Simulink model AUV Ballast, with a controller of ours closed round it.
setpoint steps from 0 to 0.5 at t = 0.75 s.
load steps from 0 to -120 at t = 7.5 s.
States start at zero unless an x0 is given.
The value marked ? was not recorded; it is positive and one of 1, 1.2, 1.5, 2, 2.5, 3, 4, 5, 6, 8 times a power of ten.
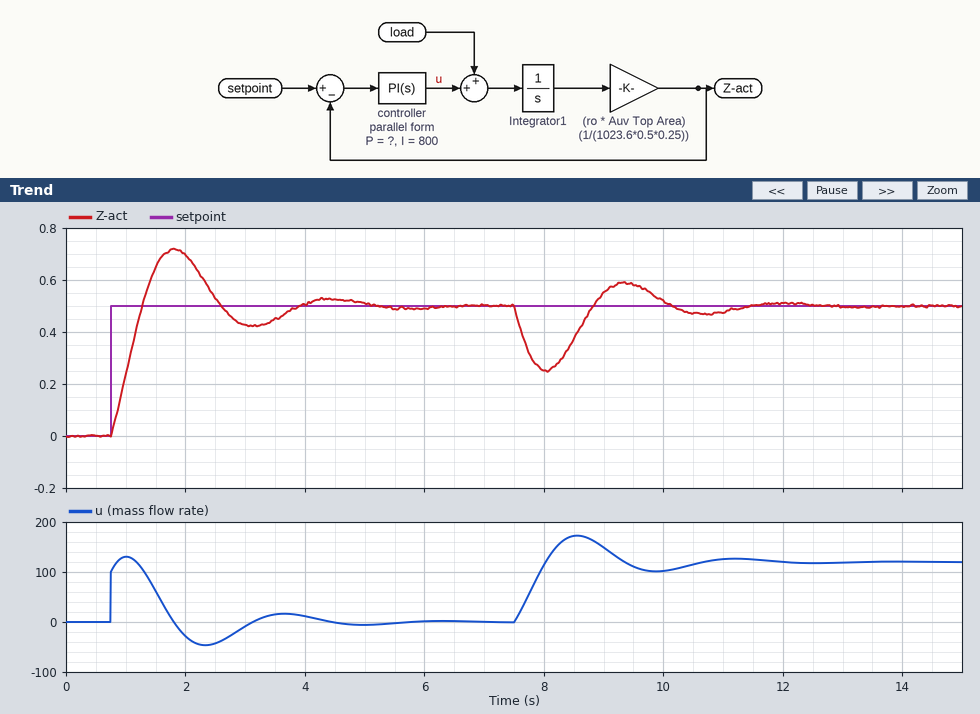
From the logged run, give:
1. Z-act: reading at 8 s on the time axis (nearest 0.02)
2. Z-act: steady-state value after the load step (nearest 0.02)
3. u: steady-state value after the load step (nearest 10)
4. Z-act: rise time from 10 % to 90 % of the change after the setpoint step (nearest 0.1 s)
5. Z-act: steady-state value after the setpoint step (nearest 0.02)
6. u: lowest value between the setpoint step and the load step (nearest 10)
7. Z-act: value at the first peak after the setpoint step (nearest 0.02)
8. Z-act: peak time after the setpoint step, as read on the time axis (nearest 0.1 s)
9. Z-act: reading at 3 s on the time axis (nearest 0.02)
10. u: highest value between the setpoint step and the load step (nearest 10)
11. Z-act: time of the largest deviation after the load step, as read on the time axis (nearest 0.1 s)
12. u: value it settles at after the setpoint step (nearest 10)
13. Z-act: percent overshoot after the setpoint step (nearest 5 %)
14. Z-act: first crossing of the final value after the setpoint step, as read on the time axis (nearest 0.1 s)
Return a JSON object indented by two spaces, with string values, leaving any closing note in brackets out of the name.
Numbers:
{
  "Z-act: reading at 8 s on the time axis": "0.26",
  "Z-act: steady-state value after the load step": "0.50",
  "u: steady-state value after the load step": "120",
  "Z-act: rise time from 10 % to 90 % of the change after the setpoint step": "0.4 s",
  "Z-act: steady-state value after the setpoint step": "0.50",
  "u: lowest value between the setpoint step and the load step": "-50",
  "Z-act: value at the first peak after the setpoint step": "0.72",
  "Z-act: peak time after the setpoint step, as read on the time axis": "1.8 s",
  "Z-act: reading at 3 s on the time axis": "0.42",
  "u: highest value between the setpoint step and the load step": "130",
  "Z-act: time of the largest deviation after the load step, as read on the time axis": "8.0 s",
  "u: value it settles at after the setpoint step": "0",
  "Z-act: percent overshoot after the setpoint step": "45 %",
  "Z-act: first crossing of the final value after the setpoint step, as read on the time axis": "1.3 s"
}
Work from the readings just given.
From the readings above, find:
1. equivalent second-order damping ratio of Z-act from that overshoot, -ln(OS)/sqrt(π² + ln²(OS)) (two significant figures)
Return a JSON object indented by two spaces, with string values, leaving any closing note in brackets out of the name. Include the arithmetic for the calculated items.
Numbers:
{
  "equivalent second-order damping ratio of Z-act from that overshoot, -ln(OS)/sqrt(π² + ln²(OS))": "ln(0.45) = -0.799; 0.799 / sqrt(9.870 + 0.638) = 0.25"
}
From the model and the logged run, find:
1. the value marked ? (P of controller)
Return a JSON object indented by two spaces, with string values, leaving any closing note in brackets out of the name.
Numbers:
{
  "the value marked ?": "200"
}
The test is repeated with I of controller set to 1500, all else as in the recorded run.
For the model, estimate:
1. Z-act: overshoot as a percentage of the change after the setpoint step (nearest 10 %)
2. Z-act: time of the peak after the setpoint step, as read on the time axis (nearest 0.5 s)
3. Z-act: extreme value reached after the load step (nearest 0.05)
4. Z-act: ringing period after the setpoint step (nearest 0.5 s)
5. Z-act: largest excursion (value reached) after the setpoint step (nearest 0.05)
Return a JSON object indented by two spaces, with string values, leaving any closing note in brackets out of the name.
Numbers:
{
  "Z-act: overshoot as a percentage of the change after the setpoint step": "50 %",
  "Z-act: time of the peak after the setpoint step, as read on the time axis": "1.5 s",
  "Z-act: extreme value reached after the load step": "0.30",
  "Z-act: ringing period after the setpoint step": "2.0 s",
  "Z-act: largest excursion (value reached) after the setpoint step": "0.75"
}
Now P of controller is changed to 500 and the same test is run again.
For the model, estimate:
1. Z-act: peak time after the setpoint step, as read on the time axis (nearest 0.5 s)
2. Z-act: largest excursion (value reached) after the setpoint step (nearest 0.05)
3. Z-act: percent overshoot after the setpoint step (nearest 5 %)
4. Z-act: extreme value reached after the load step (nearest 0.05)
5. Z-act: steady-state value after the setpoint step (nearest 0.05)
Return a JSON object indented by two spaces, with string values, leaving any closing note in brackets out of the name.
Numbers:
{
  "Z-act: peak time after the setpoint step, as read on the time axis": "1.5 s",
  "Z-act: largest excursion (value reached) after the setpoint step": "0.60",
  "Z-act: percent overshoot after the setpoint step": "20 %",
  "Z-act: extreme value reached after the load step": "0.35",
  "Z-act: steady-state value after the setpoint step": "0.50"
}
